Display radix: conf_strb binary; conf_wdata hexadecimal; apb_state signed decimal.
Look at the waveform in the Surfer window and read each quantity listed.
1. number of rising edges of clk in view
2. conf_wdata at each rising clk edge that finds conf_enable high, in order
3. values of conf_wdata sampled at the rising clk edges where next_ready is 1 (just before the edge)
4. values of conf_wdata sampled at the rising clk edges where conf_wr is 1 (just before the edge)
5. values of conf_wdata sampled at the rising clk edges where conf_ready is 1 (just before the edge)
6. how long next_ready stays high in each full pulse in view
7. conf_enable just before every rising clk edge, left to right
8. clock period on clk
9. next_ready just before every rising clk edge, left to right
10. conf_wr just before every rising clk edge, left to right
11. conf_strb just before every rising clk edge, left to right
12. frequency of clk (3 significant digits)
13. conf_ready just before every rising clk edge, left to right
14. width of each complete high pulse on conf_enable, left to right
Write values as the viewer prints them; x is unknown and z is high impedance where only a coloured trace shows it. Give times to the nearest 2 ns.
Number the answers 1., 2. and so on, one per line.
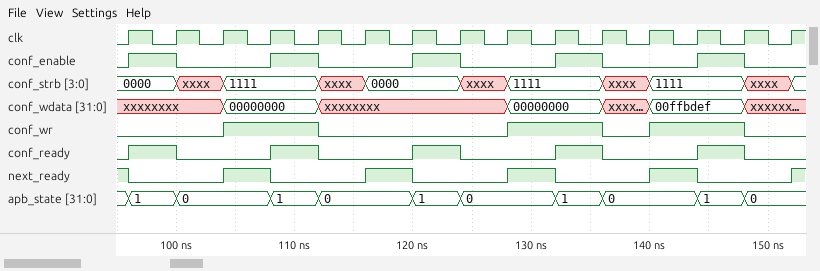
1. 15
2. xxxxxxxx, 00000000, xxxxxxxx, 00000000, 00ffbdef
3. xxxxxxxx, 00000000, xxxxxxxx, 00000000, 00ffbdef
4. 00000000, 00000000, 00000000, 00000000, 00ffbdef, 00ffbdef
5. xxxxxxxx, 00000000, xxxxxxxx, 00000000, 00ffbdef
6. 4 ns, 4 ns, 4 ns, 4 ns
7. 0 1 0 0 1 0 0 1 0 0 1 0 0 1 0
8. 4 ns
9. 1 0 0 1 0 0 1 0 0 1 0 0 1 0 0
10. 0 0 0 1 1 0 0 0 0 1 1 0 1 1 0
11. 0000, 0000, xxxx, 1111, 1111, xxxx, 0000, 0000, xxxx, 1111, 1111, xxxx, 1111, 1111, xxxx
12. 250 MHz
13. 0 1 0 0 1 0 0 1 0 0 1 0 0 1 0
14. 4 ns, 4 ns, 4 ns, 4 ns, 4 ns
